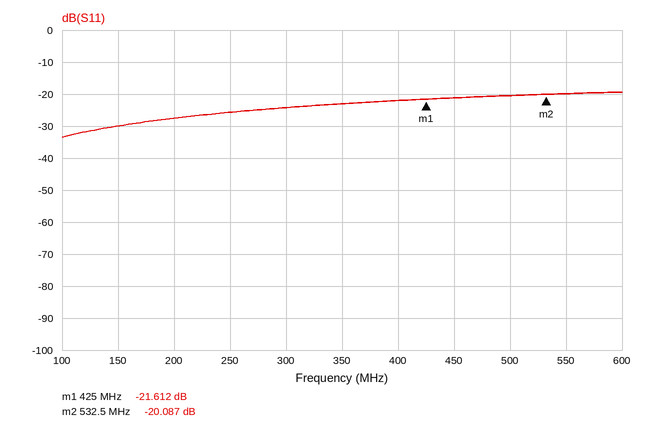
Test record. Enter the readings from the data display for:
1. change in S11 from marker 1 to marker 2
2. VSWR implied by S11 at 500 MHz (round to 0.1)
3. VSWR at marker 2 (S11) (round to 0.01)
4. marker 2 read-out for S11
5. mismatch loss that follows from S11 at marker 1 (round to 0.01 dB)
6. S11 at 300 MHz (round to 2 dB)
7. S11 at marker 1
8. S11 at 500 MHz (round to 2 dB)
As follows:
1.525 dB
1.2
1.22
-20.087 dB
0.03 dB
-24 dB
-21.612 dB
-20 dB
